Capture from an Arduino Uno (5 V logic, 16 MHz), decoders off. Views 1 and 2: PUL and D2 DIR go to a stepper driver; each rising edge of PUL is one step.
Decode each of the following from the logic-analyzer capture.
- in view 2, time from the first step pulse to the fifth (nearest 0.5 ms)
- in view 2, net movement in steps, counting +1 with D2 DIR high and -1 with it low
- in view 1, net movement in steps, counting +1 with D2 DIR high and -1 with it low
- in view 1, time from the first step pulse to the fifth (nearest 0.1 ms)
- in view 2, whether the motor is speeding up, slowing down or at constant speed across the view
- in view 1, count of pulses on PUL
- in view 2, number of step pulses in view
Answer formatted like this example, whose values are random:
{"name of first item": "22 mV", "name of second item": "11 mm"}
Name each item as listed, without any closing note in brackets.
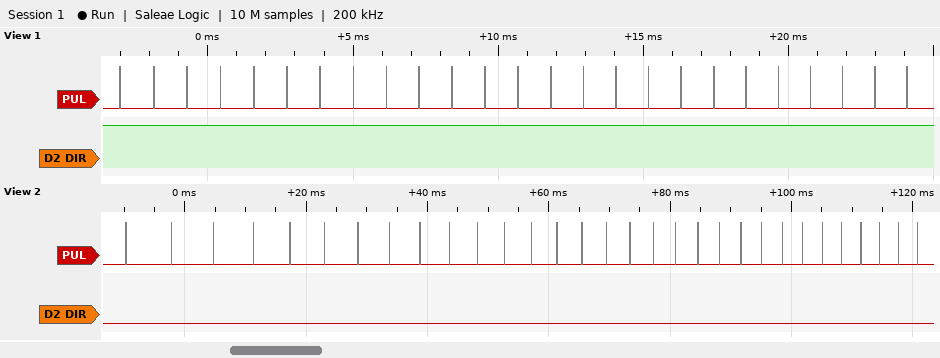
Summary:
{"in view 2, time from the first step pulse to the fifth": "27.0 ms", "in view 2, net movement in steps, counting +1 with D2 DIR high and -1 with it low": "-31", "in view 1, net movement in steps, counting +1 with D2 DIR high and -1 with it low": "+25", "in view 1, time from the first step pulse to the fifth": "4.6 ms", "in view 2, whether the motor is speeding up, slowing down or at constant speed across the view": "speeding up", "in view 1, count of pulses on PUL": "25", "in view 2, number of step pulses in view": "31"}
